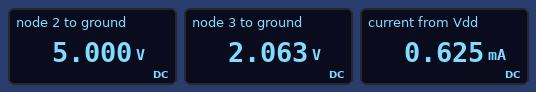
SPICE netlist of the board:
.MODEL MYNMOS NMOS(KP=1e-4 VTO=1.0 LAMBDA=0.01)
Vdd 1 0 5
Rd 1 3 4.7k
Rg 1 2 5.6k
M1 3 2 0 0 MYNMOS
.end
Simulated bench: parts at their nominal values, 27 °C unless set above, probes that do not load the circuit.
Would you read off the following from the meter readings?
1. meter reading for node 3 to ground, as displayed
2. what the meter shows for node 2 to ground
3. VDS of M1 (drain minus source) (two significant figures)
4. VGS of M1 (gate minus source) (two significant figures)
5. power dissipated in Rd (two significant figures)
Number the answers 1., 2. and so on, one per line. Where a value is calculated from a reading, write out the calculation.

1. 2.063 V
2. 5.000 V
3. 2.063 V = 2.1 V
4. 5 V = 5.0 V
5. (5 V - 2.063 V)^2 / 4.7 kΩ = 1.8 mW
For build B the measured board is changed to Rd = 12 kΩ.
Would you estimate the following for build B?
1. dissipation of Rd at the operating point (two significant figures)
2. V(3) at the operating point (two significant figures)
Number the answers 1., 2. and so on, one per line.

1. 1.4 mW
2. 950 mV
